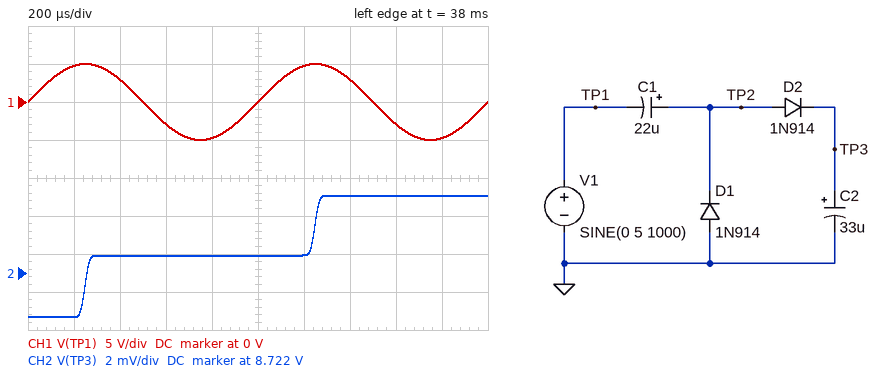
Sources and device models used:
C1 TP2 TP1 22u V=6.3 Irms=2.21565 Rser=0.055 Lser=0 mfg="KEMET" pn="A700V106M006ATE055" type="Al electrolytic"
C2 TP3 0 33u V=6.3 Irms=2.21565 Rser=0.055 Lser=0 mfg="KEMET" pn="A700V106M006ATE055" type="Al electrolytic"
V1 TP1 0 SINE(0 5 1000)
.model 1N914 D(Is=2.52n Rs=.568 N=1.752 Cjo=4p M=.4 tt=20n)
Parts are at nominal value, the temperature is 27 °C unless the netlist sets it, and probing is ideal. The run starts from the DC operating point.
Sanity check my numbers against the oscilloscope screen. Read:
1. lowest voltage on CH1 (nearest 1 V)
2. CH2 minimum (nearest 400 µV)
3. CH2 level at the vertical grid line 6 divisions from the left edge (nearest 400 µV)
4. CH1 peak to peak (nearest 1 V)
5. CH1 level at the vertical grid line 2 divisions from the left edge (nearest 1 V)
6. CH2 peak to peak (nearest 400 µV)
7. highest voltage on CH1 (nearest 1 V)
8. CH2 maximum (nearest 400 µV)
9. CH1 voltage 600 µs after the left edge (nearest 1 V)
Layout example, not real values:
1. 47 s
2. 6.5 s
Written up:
1. -5 V
2. 8.7196 V
3. 8.7228 V
4. 10 V
5. 3 V
6. 6.4 mV
7. 5 V
8. 8.7260 V
9. -3 V
